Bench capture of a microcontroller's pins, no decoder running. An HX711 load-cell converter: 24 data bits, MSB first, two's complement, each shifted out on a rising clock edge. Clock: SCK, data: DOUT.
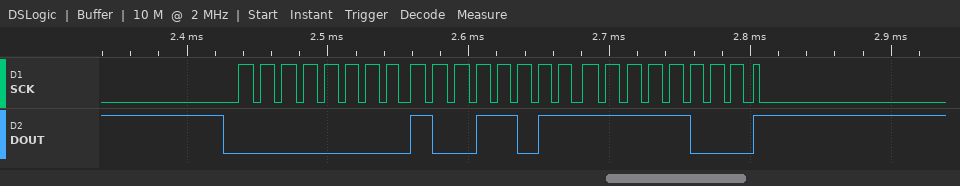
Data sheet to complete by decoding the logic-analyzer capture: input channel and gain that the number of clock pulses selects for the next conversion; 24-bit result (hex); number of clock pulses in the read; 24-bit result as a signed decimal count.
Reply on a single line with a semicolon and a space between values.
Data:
channel A, gain 128; 0x009BF8; 25; 39928
